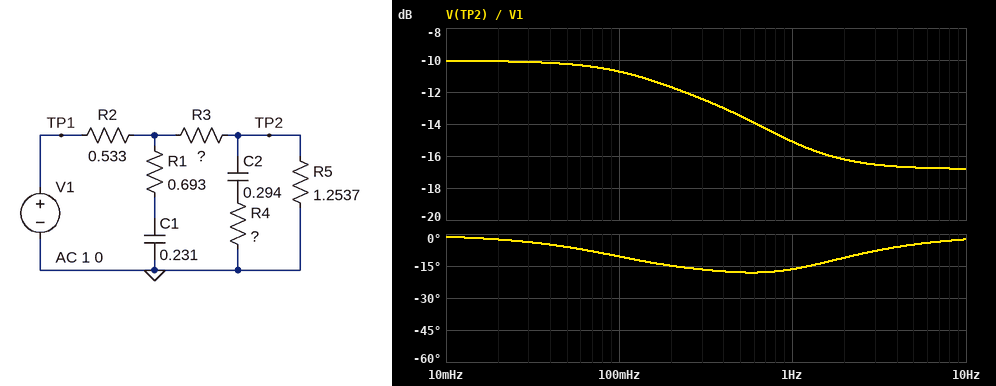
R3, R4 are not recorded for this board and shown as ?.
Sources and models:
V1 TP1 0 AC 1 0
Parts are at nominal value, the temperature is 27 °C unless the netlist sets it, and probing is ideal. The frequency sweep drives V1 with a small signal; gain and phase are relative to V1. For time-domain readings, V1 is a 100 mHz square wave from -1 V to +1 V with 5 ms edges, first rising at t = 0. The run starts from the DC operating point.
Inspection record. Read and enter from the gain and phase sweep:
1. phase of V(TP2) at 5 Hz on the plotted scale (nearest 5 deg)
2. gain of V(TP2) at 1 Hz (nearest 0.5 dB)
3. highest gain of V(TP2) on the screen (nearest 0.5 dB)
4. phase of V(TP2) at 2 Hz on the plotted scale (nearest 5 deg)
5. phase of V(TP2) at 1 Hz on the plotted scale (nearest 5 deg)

-5 deg
-15.0 dB
-10.0 dB
-10 deg
-15 deg
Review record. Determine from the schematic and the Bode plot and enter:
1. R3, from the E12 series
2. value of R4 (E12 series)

2.2 Ω
2.7 Ω
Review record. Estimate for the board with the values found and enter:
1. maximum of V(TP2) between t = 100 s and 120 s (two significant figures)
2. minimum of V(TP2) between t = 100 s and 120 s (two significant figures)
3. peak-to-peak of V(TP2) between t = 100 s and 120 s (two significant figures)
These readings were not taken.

310 mV
-310 mV
630 mV
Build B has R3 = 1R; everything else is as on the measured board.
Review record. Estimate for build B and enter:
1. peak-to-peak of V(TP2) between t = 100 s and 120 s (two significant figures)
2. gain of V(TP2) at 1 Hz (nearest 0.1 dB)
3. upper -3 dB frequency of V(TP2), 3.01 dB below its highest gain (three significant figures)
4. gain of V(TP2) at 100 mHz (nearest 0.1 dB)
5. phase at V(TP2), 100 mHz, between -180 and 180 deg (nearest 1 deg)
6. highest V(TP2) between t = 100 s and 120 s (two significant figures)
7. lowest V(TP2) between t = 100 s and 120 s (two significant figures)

900 mV
-11.4 dB
513 mHz
-7.5 dB
-9 deg
450 mV
-450 mV
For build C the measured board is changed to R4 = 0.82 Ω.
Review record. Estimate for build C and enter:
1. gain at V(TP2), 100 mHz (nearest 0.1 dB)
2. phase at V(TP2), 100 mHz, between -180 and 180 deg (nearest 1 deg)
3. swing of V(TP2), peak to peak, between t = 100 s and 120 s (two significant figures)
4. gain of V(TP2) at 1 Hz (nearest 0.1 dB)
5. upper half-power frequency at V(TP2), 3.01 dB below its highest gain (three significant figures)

-10.4 dB
-12 deg
630 mV
-17.8 dB
343 mHz
